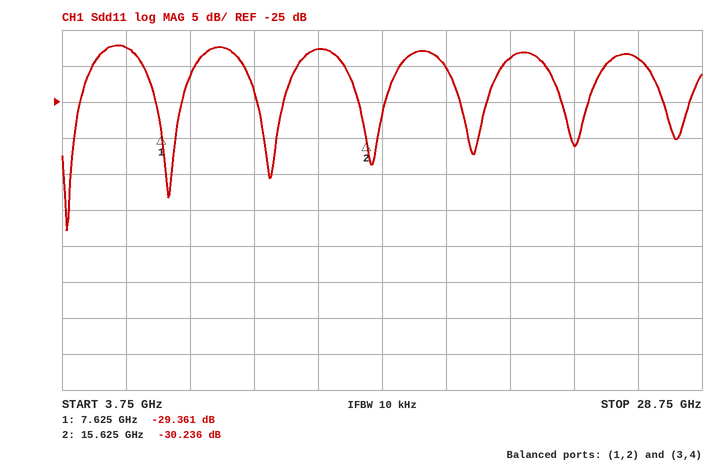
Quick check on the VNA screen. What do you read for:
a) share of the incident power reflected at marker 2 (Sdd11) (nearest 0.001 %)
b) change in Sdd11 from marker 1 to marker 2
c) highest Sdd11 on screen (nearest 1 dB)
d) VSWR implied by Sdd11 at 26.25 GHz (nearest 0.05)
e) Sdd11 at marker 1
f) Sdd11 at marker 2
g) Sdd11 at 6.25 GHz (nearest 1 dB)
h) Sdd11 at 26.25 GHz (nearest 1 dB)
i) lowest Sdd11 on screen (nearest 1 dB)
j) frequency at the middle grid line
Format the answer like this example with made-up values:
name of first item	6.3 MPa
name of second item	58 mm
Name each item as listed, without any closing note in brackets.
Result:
share of the incident power reflected at marker 2 (Sdd11)	0.095 %
change in Sdd11 from marker 1 to marker 2	-0.875 dB
highest Sdd11 on screen	-17 dB
VSWR implied by Sdd11 at 26.25 GHz	1.25
Sdd11 at marker 1	-29.361 dB
Sdd11 at marker 2	-30.236 dB
Sdd11 at 6.25 GHz	-17 dB
Sdd11 at 26.25 GHz	-19 dB
lowest Sdd11 on screen	-43 dB
frequency at the middle grid line	16.25 GHz
